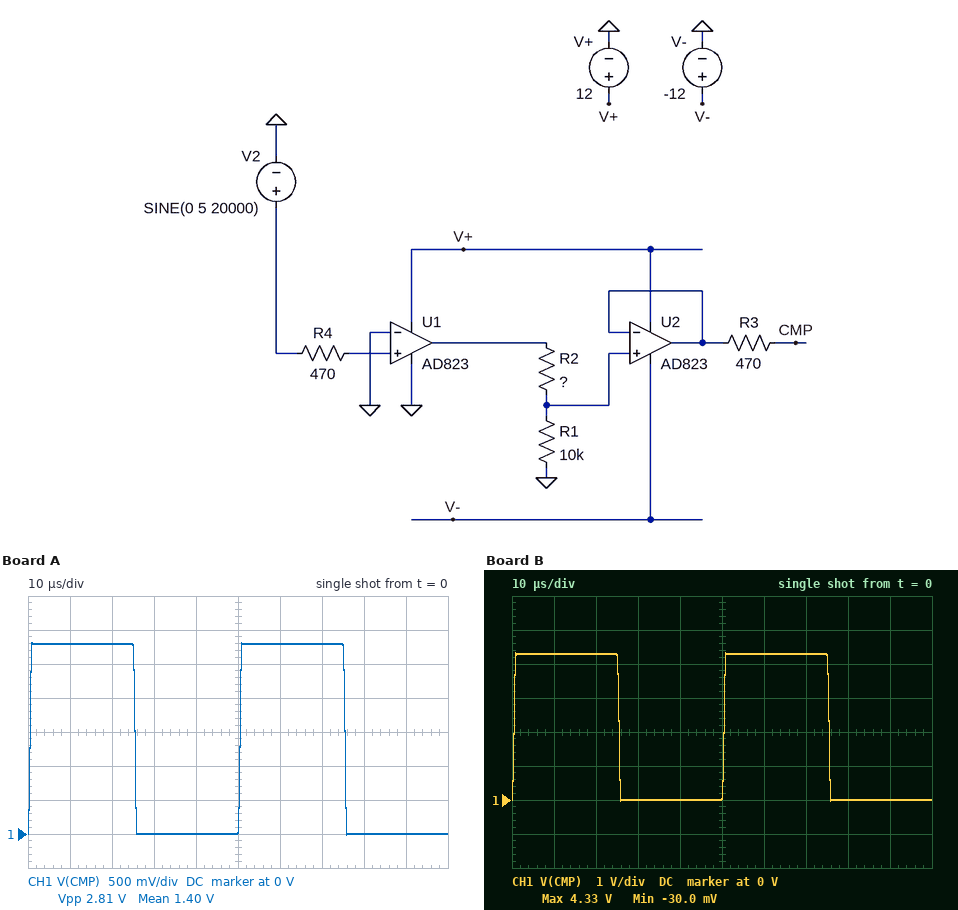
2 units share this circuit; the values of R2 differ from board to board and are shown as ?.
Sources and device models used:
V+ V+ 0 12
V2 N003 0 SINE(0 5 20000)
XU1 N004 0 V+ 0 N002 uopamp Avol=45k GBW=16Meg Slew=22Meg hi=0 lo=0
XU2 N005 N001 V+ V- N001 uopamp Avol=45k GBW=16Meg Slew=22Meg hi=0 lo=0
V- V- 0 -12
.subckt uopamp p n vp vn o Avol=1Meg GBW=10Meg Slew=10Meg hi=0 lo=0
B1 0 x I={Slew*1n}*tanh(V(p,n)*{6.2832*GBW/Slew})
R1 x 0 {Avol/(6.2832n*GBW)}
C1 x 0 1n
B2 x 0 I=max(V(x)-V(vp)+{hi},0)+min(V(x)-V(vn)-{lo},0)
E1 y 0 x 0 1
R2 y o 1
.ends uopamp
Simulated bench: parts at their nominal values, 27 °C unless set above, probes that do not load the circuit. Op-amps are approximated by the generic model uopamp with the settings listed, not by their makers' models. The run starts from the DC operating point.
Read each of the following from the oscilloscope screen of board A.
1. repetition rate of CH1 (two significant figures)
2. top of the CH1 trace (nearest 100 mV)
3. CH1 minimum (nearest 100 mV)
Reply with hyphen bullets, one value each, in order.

- 20 kHz
- 2.8 V
- 0 V
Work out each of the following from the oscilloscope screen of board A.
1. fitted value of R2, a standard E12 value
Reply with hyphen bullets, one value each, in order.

- 33 kΩ
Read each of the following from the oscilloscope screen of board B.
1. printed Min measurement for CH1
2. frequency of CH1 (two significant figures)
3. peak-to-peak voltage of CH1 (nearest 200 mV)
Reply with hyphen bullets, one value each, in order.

- -30.0 mV
- 20 kHz
- 4.4 V
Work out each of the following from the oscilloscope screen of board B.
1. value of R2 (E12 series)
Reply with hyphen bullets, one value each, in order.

- 18 kΩ
